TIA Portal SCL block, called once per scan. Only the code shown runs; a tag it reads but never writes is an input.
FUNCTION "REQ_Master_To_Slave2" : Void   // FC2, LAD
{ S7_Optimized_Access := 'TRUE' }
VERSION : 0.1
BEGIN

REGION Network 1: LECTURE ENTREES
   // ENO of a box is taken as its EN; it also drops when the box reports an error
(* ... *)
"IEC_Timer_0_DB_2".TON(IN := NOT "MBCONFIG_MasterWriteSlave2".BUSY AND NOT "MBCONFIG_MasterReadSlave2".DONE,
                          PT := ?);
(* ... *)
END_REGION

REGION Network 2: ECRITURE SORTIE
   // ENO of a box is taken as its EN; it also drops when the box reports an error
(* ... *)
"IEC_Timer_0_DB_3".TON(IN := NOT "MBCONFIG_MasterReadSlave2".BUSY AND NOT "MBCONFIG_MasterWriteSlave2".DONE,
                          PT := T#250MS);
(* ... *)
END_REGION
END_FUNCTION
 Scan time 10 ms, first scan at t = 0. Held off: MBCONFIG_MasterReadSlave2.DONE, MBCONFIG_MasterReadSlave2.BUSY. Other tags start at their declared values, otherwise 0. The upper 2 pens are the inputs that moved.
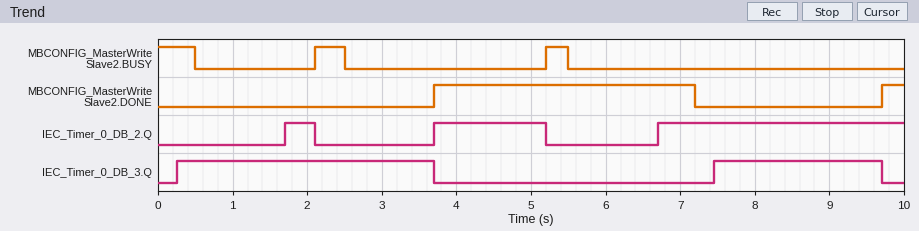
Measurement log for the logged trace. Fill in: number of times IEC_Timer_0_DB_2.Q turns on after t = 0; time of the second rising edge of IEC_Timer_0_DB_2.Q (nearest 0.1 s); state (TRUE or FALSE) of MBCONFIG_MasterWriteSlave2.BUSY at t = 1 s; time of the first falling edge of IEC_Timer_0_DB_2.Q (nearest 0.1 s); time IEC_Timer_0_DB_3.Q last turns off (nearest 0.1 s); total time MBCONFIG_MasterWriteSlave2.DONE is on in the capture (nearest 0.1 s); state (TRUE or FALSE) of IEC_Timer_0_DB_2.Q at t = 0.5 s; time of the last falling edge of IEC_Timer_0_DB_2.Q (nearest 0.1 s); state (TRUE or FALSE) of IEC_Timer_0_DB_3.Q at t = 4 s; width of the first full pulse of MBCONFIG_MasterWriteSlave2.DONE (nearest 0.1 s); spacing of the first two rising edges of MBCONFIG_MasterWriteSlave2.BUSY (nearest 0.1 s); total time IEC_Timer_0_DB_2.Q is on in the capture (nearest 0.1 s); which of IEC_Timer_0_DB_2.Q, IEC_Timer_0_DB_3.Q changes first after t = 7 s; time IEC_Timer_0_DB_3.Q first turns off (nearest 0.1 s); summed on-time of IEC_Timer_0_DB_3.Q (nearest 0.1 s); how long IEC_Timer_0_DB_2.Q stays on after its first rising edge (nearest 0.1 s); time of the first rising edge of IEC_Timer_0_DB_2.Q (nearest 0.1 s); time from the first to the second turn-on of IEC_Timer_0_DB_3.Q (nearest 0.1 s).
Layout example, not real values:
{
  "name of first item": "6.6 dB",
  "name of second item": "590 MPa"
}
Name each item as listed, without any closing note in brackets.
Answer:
{
  "number of times IEC_Timer_0_DB_2.Q turns on after t = 0": "3",
  "time of the second rising edge of IEC_Timer_0_DB_2.Q": "3.7 s",
  "state (TRUE or FALSE) of MBCONFIG_MasterWriteSlave2.BUSY at t = 1 s": "FALSE",
  "time of the first falling edge of IEC_Timer_0_DB_2.Q": "2.1 s",
  "time IEC_Timer_0_DB_3.Q last turns off": "9.7 s",
  "total time MBCONFIG_MasterWriteSlave2.DONE is on in the capture": "3.8 s",
  "state (TRUE or FALSE) of IEC_Timer_0_DB_2.Q at t = 0.5 s": "FALSE",
  "time of the last falling edge of IEC_Timer_0_DB_2.Q": "5.2 s",
  "state (TRUE or FALSE) of IEC_Timer_0_DB_3.Q at t = 4 s": "FALSE",
  "width of the first full pulse of MBCONFIG_MasterWriteSlave2.DONE": "3.5 s",
  "spacing of the first two rising edges of MBCONFIG_MasterWriteSlave2.BUSY": "3.1 s",
  "total time IEC_Timer_0_DB_2.Q is on in the capture": "5.2 s",
  "which of IEC_Timer_0_DB_2.Q, IEC_Timer_0_DB_3.Q changes first after t = 7 s": "IEC_Timer_0_DB_3.Q",
  "time IEC_Timer_0_DB_3.Q first turns off": "3.7 s",
  "summed on-time of IEC_Timer_0_DB_3.Q": "5.7 s",
  "how long IEC_Timer_0_DB_2.Q stays on after its first rising edge": "0.4 s",
  "time of the first rising edge of IEC_Timer_0_DB_2.Q": "1.7 s",
  "time from the first to the second turn-on of IEC_Timer_0_DB_3.Q": "7.2 s"
}
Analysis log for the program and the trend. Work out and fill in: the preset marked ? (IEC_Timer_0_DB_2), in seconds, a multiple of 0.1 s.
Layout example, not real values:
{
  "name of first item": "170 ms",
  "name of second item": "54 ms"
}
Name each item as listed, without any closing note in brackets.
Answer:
{
  "the preset marked ? (IEC_Timer_0_DB_2), in seconds, a multiple of 0.1 s": "1.2 s"
}
